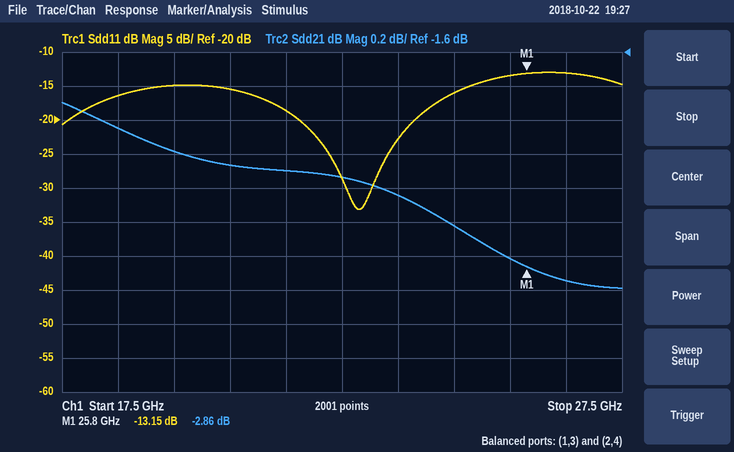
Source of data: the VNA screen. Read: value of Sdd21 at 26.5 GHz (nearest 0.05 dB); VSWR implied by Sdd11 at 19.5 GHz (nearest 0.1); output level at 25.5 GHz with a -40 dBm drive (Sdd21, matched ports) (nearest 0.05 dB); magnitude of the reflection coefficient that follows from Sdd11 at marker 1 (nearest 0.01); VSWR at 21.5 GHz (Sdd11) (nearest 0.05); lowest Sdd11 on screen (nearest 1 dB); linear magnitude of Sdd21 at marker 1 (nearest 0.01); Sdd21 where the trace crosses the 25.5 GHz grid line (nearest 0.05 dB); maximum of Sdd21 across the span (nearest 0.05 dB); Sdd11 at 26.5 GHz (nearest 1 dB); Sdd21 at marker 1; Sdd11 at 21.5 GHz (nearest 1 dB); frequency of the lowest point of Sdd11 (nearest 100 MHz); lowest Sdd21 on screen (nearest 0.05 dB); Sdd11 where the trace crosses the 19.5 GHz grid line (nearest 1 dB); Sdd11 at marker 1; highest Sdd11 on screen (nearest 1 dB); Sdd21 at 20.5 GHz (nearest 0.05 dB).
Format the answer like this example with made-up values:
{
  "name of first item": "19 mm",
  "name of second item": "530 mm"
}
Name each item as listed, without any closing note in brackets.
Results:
{
  "value of Sdd21 at 26.5 GHz": "-2.95 dB",
  "VSWR implied by Sdd11 at 19.5 GHz": "1.4",
  "output level at 25.5 GHz with a -40 dBm drive (Sdd21, matched ports)": "-42.80 dBm",
  "magnitude of the reflection coefficient that follows from Sdd11 at marker 1": "0.22",
  "VSWR at 21.5 GHz (Sdd11)": "1.25",
  "lowest Sdd11 on screen": "-33 dB",
  "linear magnitude of Sdd21 at marker 1": "0.72",
  "Sdd21 where the trace crosses the 25.5 GHz grid line": "-2.80 dB",
  "maximum of Sdd21 across the span": "-1.90 dB",
  "Sdd11 at 26.5 GHz": "-13 dB",
  "Sdd21 at marker 1": "-2.86 dB",
  "Sdd11 at 21.5 GHz": "-19 dB",
  "frequency of the lowest point of Sdd11": "22.8 GHz",
  "lowest Sdd21 on screen": "-3.00 dB",
  "Sdd11 where the trace crosses the 19.5 GHz grid line": "-15 dB",
  "Sdd11 at marker 1": "-13.15 dB",
  "highest Sdd11 on screen": "-13 dB",
  "Sdd21 at 20.5 GHz": "-2.25 dB"
}
